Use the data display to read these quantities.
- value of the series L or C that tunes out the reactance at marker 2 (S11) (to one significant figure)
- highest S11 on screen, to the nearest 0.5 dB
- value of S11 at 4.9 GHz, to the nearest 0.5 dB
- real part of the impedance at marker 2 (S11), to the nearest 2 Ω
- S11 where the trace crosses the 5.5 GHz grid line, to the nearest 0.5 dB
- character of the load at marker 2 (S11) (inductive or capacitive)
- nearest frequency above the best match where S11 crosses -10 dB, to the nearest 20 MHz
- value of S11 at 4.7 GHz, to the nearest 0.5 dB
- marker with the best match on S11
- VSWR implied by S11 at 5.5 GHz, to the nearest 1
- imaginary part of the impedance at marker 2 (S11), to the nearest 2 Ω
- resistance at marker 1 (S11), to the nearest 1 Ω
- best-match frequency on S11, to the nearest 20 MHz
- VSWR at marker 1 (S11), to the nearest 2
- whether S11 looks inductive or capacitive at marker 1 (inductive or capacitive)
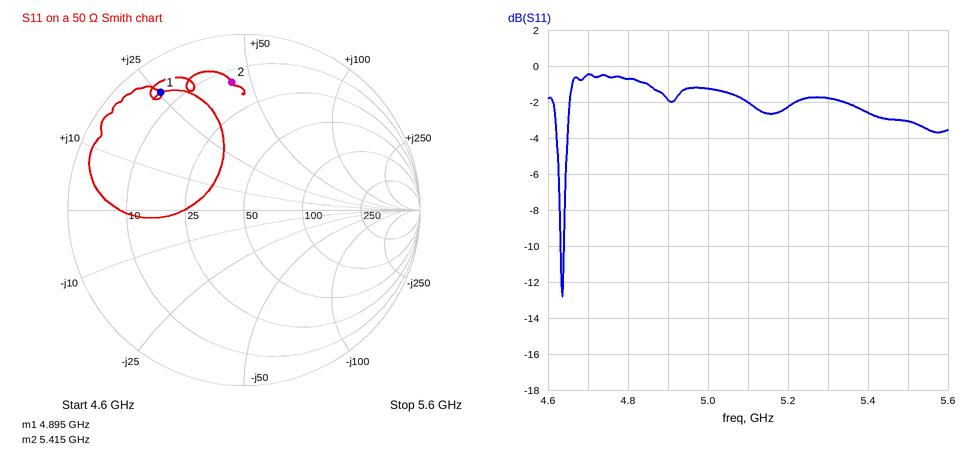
700 fF
-0.5 dB
-2.0 dB
14 Ω
-3.0 dB
inductive
4.64 GHz
-0.5 dB
marker 2
6
+44 Ω
6 Ω
4.64 GHz
10
inductive
